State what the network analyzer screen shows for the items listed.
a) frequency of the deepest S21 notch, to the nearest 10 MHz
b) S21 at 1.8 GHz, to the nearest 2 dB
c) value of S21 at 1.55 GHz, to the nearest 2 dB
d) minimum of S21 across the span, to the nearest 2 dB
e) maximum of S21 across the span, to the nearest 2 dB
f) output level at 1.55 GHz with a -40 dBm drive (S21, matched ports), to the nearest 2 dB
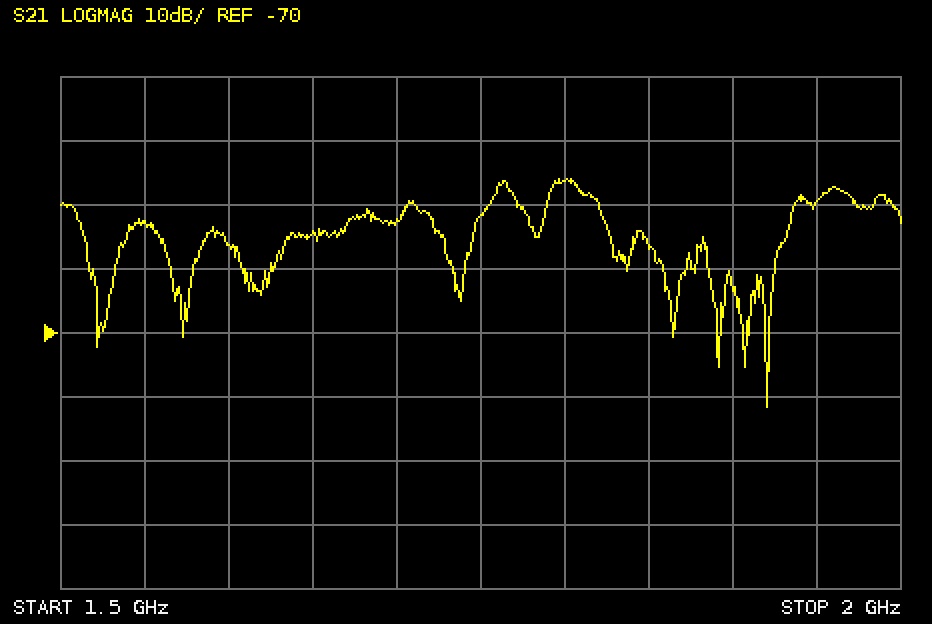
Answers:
1.92 GHz
-46 dB
-52 dB
-82 dB
-46 dB
-92 dBm
